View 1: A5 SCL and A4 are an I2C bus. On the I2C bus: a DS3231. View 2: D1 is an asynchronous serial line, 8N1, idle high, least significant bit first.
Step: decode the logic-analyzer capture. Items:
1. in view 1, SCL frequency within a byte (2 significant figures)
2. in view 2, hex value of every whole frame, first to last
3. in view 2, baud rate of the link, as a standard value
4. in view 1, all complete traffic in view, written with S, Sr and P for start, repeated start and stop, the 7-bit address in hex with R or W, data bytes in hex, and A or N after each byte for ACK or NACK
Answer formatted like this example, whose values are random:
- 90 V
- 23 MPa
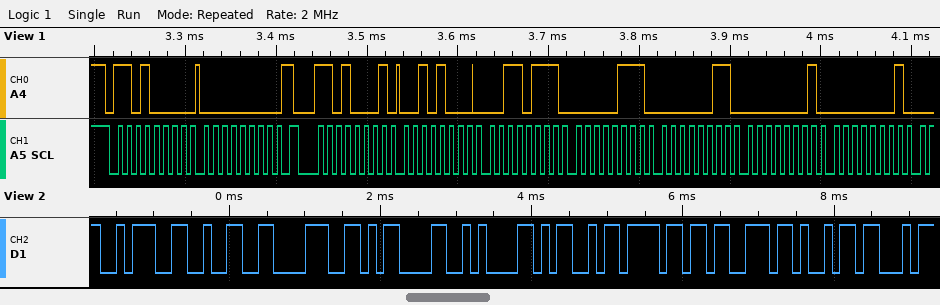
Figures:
- 100 kHz
- 0x3A 0x32 0x38 0x0D 0x0A 0x4D 0x6F 0x73 0x69
- 9600 baud
- S 68W A 00 A Sr 68R A 28 A 37 A 07 A 03 A 01 A 01 A
